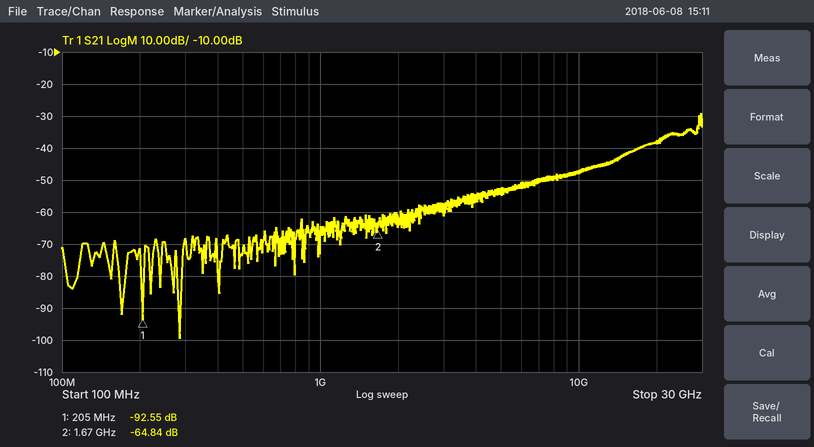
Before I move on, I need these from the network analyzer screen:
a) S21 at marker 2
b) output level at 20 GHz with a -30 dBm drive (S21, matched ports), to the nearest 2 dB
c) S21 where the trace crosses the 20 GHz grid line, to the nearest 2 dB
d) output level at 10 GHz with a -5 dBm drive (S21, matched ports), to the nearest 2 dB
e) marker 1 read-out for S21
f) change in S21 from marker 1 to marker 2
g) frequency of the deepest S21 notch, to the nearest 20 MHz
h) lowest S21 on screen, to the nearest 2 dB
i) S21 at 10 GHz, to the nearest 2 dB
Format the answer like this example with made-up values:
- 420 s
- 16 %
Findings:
- -64.84 dB
- -68 dBm
- -38 dB
- -52 dBm
- -92.55 dB
- 27.71 dB
- 280 MHz
- -100 dB
- -48 dB
